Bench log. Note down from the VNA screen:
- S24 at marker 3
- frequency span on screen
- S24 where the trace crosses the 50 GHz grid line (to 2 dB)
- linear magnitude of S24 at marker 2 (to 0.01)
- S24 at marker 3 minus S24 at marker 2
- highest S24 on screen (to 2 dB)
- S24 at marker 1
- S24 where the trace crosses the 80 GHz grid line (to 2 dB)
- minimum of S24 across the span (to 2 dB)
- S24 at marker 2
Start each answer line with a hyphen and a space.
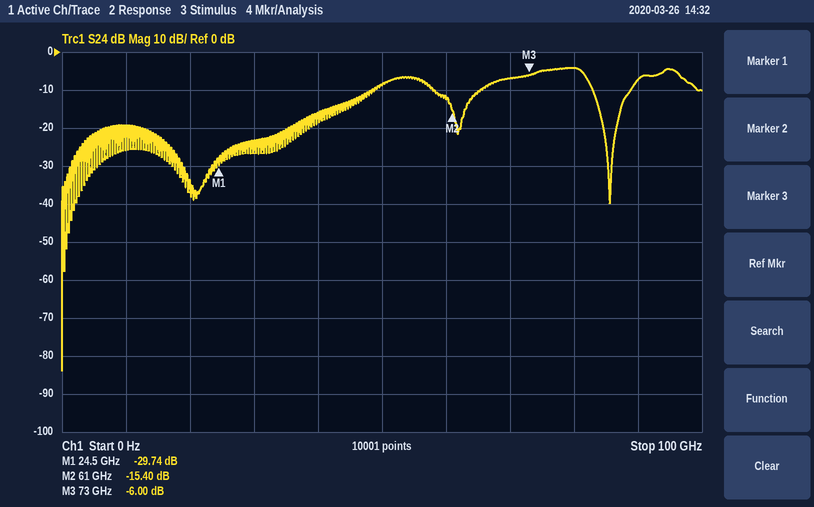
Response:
- -6.00 dB
- 100 GHz
- -8 dB
- 0.17
- 9.40 dB
- -4 dB
- -29.74 dB
- -4 dB
- -84 dB
- -15.40 dB
